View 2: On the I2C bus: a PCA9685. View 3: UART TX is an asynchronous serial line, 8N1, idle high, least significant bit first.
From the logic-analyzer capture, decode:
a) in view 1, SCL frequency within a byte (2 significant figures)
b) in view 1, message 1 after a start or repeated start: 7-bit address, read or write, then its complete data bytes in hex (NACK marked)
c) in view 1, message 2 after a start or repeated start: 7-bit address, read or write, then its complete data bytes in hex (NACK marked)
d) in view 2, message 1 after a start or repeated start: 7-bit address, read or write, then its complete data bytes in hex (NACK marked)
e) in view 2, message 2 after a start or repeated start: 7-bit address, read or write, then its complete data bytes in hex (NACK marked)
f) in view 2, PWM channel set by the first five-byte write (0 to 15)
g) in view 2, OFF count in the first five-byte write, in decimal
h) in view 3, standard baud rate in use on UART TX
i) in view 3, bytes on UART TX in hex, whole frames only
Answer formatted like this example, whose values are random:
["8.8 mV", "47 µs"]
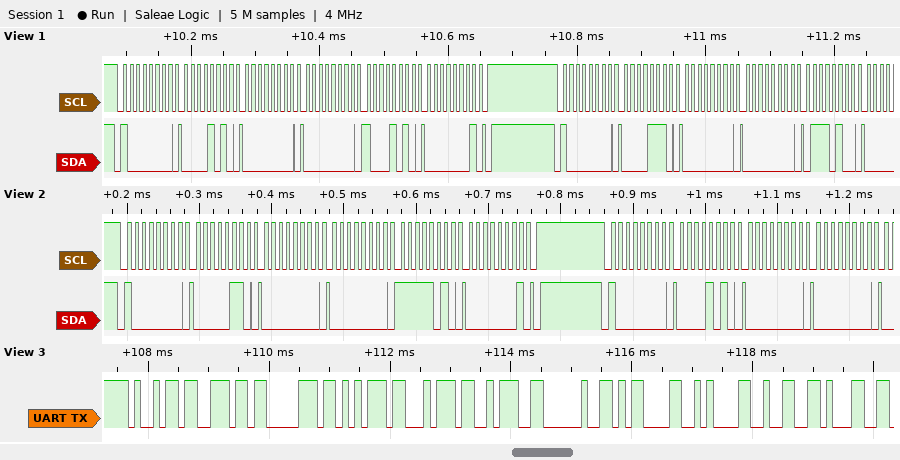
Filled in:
["100 kHz", "0x40 write: 0A 00 00 8A 01", "0x40 write: 0E 00 00 74", "0x40 write: 06 00 00 FA 01", "0x40 write: 0A 00 00", "0", "506", "9600 baud", "69 6E 70 75 74 3A 20 0D 0A 32 31"]
